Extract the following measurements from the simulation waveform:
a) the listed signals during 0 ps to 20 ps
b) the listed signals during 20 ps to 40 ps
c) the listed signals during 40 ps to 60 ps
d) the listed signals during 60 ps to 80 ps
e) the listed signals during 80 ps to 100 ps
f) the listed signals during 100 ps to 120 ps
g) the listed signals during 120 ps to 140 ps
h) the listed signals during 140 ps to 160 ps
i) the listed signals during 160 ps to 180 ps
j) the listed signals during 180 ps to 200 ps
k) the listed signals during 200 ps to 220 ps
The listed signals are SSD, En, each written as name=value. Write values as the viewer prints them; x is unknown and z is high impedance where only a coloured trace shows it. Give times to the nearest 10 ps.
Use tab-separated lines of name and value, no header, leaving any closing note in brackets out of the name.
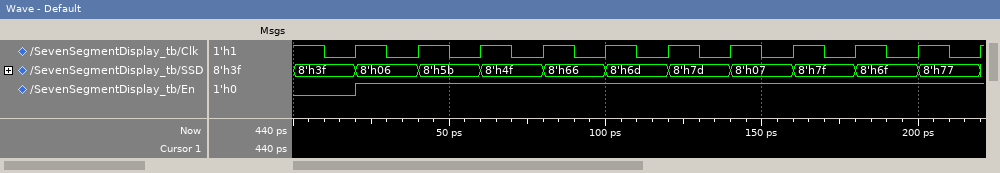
the listed signals during 0 ps to 20 ps	SSD=8'h3f, En=0
the listed signals during 20 ps to 40 ps	SSD=8'h06, En=1
the listed signals during 40 ps to 60 ps	SSD=8'h5b, En=1
the listed signals during 60 ps to 80 ps	SSD=8'h4f, En=1
the listed signals during 80 ps to 100 ps	SSD=8'h66, En=1
the listed signals during 100 ps to 120 ps	SSD=8'h6d, En=1
the listed signals during 120 ps to 140 ps	SSD=8'h7d, En=1
the listed signals during 140 ps to 160 ps	SSD=8'h07, En=1
the listed signals during 160 ps to 180 ps	SSD=8'h7f, En=1
the listed signals during 180 ps to 200 ps	SSD=8'h6f, En=1
the listed signals during 200 ps to 220 ps	SSD=8'h77, En=1
